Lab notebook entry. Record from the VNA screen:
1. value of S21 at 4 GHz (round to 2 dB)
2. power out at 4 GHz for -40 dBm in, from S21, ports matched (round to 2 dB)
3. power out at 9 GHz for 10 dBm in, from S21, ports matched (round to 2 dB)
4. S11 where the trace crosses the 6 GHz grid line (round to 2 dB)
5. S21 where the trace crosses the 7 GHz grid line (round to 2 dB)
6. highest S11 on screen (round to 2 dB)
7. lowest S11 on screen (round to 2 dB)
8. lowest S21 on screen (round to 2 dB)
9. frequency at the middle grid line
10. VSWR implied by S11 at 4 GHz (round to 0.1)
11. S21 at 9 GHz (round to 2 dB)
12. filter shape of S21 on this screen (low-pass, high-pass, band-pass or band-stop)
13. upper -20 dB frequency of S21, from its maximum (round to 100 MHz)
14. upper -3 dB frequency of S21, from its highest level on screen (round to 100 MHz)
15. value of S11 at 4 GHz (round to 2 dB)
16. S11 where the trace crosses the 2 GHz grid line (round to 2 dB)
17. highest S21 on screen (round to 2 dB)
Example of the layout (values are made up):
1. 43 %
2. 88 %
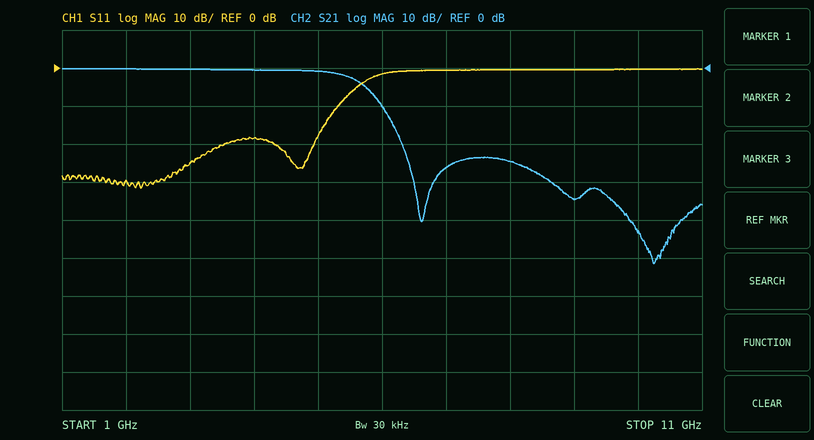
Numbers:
1. 0 dB
2. -40 dBm
3. -24 dBm
4. -2 dB
5. -26 dB
6. 0 dB
7. -32 dB
8. -52 dB
9. 6 GHz
10. 1.3
11. -34 dB
12. low-pass
13. 6.3 GHz
14. 5.6 GHz
15. -18 dB
16. -30 dB
17. 0 dB
